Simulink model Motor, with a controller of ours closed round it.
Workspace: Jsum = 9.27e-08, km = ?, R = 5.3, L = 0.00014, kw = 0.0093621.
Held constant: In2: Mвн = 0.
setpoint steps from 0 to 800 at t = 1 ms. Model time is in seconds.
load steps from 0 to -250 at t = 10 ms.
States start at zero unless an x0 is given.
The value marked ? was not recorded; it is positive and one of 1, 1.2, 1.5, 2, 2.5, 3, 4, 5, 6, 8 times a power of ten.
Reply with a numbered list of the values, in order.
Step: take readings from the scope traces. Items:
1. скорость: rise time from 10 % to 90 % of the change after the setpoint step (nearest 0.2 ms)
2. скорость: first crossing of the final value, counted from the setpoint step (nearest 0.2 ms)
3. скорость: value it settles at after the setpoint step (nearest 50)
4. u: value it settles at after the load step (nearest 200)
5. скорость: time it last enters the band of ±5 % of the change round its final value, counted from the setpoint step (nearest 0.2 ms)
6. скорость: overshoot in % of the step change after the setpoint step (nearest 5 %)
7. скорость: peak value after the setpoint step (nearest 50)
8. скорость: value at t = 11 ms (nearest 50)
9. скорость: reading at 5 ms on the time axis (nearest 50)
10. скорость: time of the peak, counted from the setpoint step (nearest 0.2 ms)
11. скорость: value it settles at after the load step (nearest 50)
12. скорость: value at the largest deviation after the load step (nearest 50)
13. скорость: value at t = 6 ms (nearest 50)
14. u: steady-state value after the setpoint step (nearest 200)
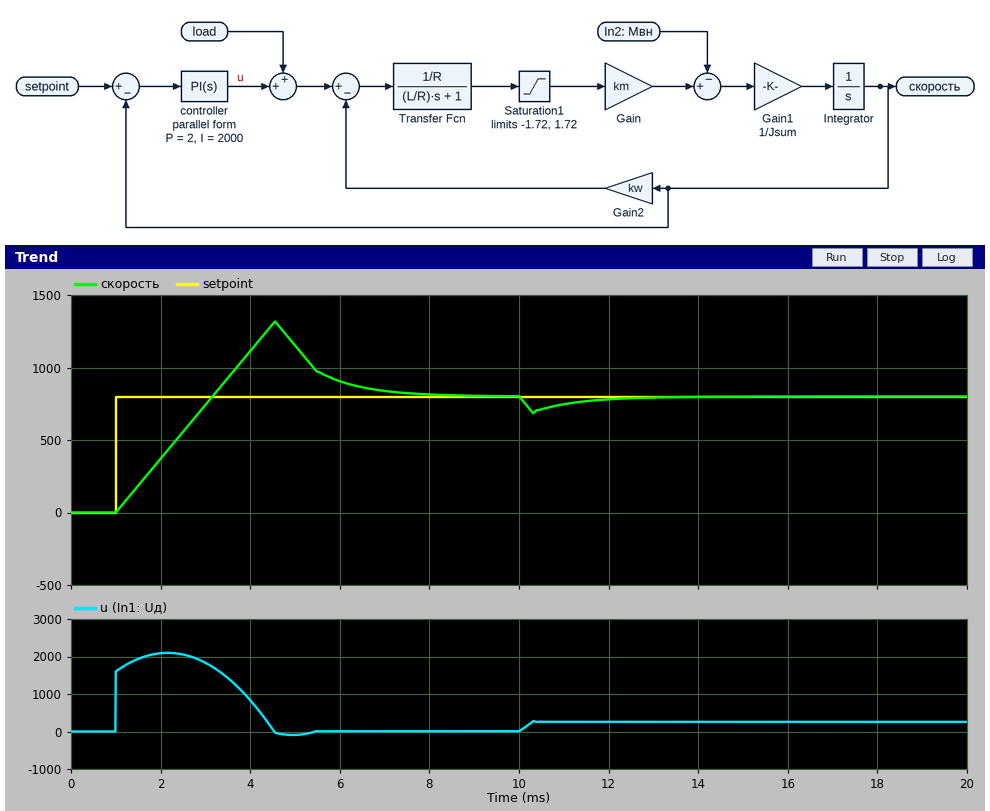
1. 1.8 ms
2. 2.2 ms
3. 800
4. 200
5. 6.0 ms
6. 65 %
7. 1300
8. 750
9. 1150
10. 3.6 ms
11. 800
12. 700
13. 900
14. 0
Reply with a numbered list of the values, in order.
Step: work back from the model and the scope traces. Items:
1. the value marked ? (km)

1. 0.02
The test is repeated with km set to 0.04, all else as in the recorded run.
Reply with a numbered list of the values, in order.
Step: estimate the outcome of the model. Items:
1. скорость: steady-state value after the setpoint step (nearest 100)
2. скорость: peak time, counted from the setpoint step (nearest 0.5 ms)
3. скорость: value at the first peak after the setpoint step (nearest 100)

1. 800
2. 1.5 ms
3. 1200
